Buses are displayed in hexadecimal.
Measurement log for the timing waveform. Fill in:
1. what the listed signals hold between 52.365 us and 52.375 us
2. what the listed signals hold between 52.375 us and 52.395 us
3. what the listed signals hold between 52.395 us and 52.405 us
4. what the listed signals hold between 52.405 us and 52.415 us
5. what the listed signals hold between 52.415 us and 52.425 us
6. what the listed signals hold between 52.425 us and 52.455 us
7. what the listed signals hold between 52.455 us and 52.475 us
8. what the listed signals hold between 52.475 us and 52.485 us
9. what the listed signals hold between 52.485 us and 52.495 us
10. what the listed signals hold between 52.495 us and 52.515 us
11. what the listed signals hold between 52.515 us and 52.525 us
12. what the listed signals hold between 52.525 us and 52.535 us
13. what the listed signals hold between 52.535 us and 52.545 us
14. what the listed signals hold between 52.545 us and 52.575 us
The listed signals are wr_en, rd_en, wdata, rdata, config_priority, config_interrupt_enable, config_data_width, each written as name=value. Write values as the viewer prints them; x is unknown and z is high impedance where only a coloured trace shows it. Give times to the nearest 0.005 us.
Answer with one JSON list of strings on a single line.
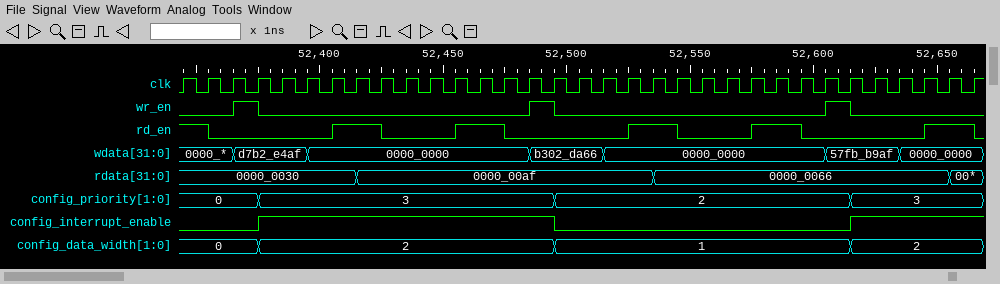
["wr_en=1, rd_en=0, wdata=d7b2_e4af, rdata=0000_0030, config_priority=0, config_interrupt_enable=0, config_data_width=0", "wr_en=0, rd_en=0, wdata=d7b2_e4af, rdata=0000_0030, config_priority=3, config_interrupt_enable=1, config_data_width=2", "wr_en=0, rd_en=0, wdata=0000_0000, rdata=0000_0030, config_priority=3, config_interrupt_enable=1, config_data_width=2", "wr_en=0, rd_en=1, wdata=0000_0000, rdata=0000_0030, config_priority=3, config_interrupt_enable=1, config_data_width=2", "wr_en=0, rd_en=1, wdata=0000_0000, rdata=0000_00af, config_priority=3, config_interrupt_enable=1, config_data_width=2", "wr_en=0, rd_en=0, wdata=0000_0000, rdata=0000_00af, config_priority=3, config_interrupt_enable=1, config_data_width=2", "wr_en=0, rd_en=1, wdata=0000_0000, rdata=0000_00af, config_priority=3, config_interrupt_enable=1, config_data_width=2", "wr_en=0, rd_en=0, wdata=0000_0000, rdata=0000_00af, config_priority=3, config_interrupt_enable=1, config_data_width=2", "wr_en=1, rd_en=0, wdata=b302_da66, rdata=0000_00af, config_priority=3, config_interrupt_enable=1, config_data_width=2", "wr_en=0, rd_en=0, wdata=b302_da66, rdata=0000_00af, config_priority=2, config_interrupt_enable=0, config_data_width=1", "wr_en=0, rd_en=0, wdata=0000_0000, rdata=0000_00af, config_priority=2, config_interrupt_enable=0, config_data_width=1", "wr_en=0, rd_en=1, wdata=0000_0000, rdata=0000_00af, config_priority=2, config_interrupt_enable=0, config_data_width=1", "wr_en=0, rd_en=1, wdata=0000_0000, rdata=0000_0066, config_priority=2, config_interrupt_enable=0, config_data_width=1", "wr_en=0, rd_en=0, wdata=0000_0000, rdata=0000_0066, config_priority=2, config_interrupt_enable=0, config_data_width=1"]
